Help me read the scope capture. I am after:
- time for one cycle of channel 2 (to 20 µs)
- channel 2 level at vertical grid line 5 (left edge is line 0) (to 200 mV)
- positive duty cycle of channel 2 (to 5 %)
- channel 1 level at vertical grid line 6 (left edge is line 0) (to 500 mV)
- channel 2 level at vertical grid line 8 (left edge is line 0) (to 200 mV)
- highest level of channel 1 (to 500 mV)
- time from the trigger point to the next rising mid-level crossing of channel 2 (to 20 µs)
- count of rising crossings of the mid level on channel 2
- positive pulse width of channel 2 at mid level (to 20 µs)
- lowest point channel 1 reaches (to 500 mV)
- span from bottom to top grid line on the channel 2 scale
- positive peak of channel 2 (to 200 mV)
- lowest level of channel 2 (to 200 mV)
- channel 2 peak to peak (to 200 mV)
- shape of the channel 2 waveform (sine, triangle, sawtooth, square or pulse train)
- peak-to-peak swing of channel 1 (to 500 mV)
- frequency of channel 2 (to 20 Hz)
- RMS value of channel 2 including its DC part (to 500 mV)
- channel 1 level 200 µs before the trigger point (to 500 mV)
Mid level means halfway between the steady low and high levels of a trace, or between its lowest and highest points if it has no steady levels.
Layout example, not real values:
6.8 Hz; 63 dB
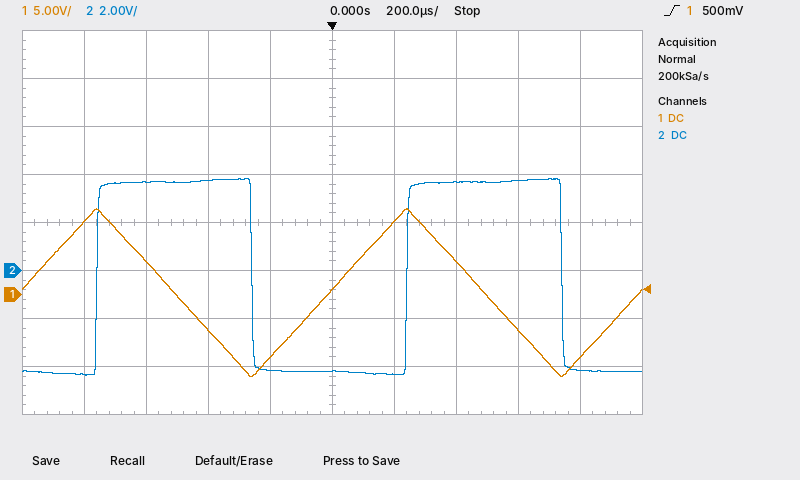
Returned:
1.00 ms; -4.2 V; 50 %; 7.5 V; 3.8 V; 9.0 V; 240 µs; 2; 500 µs; -8.5 V; 16 V; 3.8 V; -4.4 V; 8.2 V; square; 17.5 V; 1.00 kHz; 4.0 V; -6.5 V
